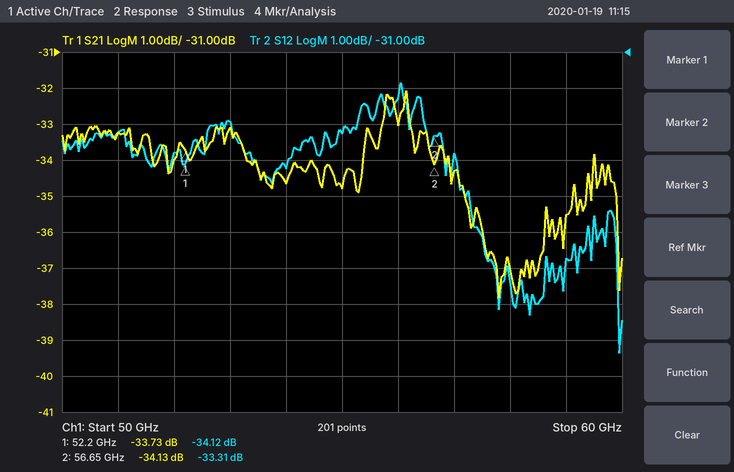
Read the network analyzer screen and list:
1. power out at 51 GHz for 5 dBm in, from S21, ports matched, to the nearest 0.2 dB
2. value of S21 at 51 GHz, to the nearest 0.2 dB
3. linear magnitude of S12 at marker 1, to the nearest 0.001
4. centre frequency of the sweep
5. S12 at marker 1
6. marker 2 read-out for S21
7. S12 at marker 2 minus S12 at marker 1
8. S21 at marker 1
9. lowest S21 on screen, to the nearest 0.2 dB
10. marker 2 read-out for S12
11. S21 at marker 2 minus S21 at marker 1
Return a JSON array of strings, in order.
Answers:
["-28.2 dBm", "-33.2 dB", "0.020", "55 GHz", "-34.12 dB", "-34.13 dB", "0.81 dB", "-33.73 dB", "-37.8 dB", "-33.31 dB", "-0.40 dB"]
